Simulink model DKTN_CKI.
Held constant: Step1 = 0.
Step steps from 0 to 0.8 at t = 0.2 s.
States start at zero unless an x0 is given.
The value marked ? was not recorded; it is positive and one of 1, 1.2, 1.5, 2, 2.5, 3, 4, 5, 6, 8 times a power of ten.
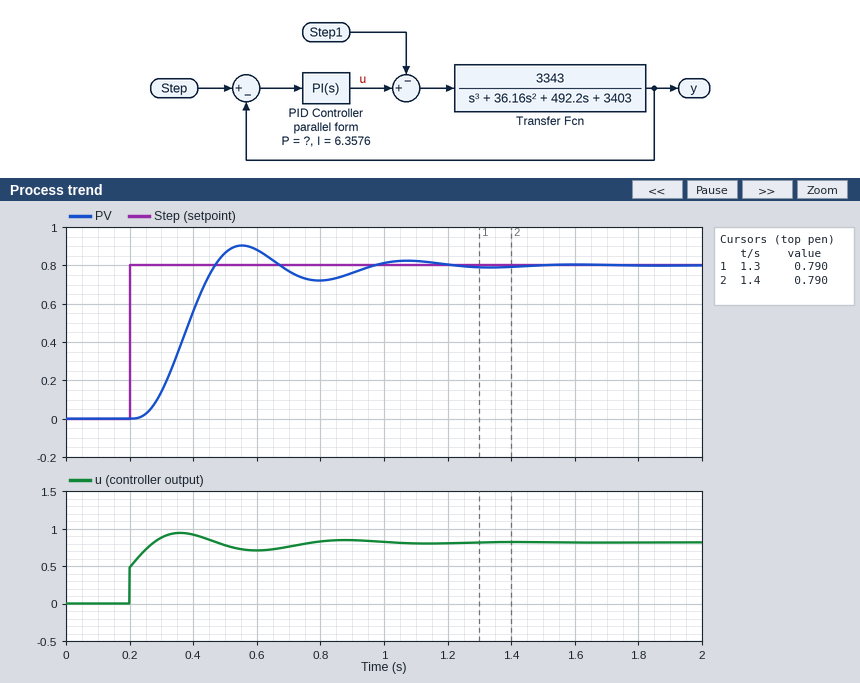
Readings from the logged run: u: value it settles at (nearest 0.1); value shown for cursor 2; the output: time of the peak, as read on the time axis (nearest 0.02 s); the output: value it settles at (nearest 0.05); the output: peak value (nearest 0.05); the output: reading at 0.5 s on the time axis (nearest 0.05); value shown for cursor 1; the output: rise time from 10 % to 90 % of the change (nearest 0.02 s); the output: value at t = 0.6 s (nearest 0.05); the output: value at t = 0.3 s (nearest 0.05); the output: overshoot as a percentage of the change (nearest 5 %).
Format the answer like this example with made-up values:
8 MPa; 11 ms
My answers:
0.8; 0.790; 0.56 s; 0.80; 0.90; 0.85; 0.790; 0.16 s; 0.90; 0.15; 15 %
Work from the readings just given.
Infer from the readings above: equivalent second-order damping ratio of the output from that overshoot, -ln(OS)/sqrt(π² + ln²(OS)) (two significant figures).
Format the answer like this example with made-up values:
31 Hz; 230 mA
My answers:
0.52
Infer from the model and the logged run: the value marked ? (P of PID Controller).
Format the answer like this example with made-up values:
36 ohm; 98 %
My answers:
0.6
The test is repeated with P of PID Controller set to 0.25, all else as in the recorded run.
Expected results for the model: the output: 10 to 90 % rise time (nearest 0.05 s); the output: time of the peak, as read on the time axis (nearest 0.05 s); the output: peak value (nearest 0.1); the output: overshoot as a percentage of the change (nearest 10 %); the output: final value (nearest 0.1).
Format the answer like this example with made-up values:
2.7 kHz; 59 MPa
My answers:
0.20 s; 0.65 s; 1.0; 20 %; 0.8
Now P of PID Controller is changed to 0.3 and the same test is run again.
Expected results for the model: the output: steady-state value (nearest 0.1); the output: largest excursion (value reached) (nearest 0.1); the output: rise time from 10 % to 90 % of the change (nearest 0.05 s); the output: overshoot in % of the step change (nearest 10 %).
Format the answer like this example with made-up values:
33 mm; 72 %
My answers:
0.8; 1.0; 0.20 s; 20 %
